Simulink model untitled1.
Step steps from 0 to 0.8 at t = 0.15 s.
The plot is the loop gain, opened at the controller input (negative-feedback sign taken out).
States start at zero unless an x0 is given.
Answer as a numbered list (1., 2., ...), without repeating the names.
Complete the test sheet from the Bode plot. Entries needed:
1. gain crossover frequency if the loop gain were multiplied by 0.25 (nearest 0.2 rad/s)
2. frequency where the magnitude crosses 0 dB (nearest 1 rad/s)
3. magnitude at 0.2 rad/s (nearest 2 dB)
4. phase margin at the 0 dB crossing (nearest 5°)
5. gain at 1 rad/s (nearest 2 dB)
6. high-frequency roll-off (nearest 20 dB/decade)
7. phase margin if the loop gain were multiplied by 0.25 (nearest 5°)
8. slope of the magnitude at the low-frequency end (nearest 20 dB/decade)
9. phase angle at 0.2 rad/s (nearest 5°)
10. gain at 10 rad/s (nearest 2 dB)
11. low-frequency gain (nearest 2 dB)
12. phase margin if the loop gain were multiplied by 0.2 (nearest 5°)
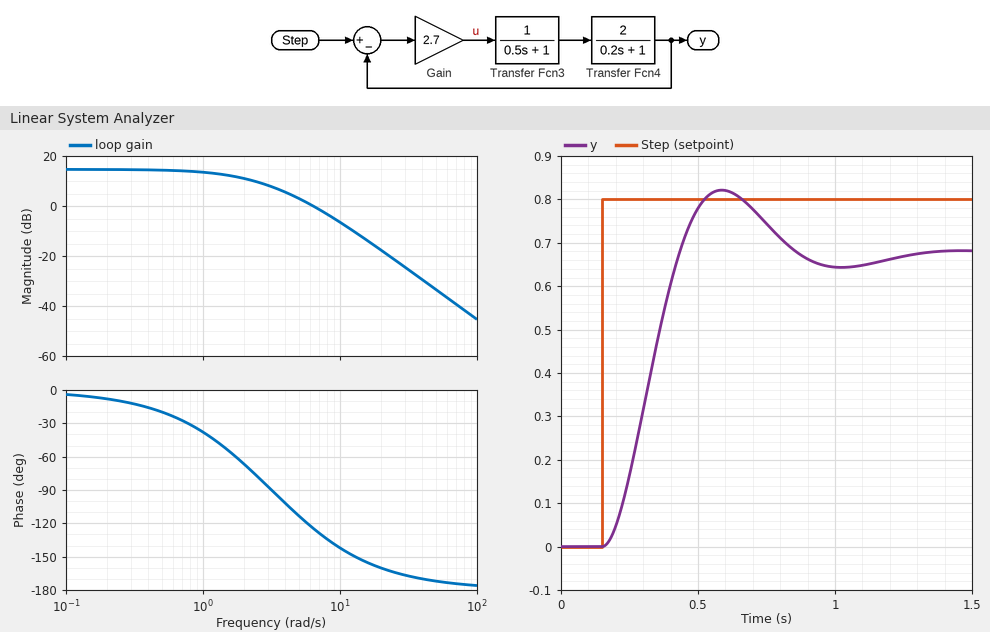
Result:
1. 1.6 rad/s
2. 6 rad/s
3. 14 dB
4. 55°
5. 14 dB
6. -40 dB/decade
7. 125°
8. 0 dB/decade
9. -10°
10. -6 dB
11. 14 dB
12. 150°
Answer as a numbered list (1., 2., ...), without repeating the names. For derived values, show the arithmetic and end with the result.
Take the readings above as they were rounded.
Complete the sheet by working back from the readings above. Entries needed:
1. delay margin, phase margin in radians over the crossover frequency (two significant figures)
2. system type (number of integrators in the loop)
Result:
1. 55 × π / 180 / 6 = 0.16 s
2. 0
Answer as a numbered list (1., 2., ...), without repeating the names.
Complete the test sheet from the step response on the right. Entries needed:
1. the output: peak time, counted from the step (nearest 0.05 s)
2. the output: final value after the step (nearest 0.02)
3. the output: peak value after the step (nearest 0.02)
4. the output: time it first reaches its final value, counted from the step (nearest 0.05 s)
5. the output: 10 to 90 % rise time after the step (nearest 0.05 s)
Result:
1. 0.45 s
2. 0.68
3. 0.82
4. 0.30 s
5. 0.20 s
